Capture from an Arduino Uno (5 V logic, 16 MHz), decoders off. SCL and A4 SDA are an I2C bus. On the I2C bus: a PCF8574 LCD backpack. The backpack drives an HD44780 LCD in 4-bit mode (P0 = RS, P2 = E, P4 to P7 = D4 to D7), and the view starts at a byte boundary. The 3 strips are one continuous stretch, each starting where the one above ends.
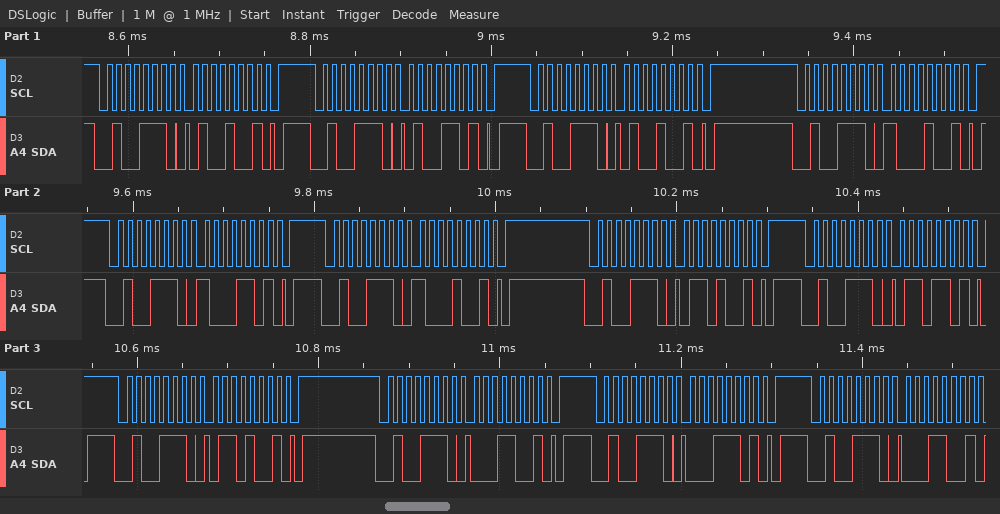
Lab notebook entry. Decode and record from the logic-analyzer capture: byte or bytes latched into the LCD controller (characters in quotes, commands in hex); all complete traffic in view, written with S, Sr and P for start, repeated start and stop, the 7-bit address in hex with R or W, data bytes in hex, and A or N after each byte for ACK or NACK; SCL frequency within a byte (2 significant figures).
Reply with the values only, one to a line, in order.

'H' 'a'
S 27W A 49 A P S 27W A 4D A P S 27W A 49 A P S 27W A 89 A P S 27W A 8D A P S 27W A 89 A P S 27W A 69 A P S 27W A 6D A P S 27W A 69 A P S 27W A 19 A P S 27W A 1D A P S 27W A 19 A
100 kHz
